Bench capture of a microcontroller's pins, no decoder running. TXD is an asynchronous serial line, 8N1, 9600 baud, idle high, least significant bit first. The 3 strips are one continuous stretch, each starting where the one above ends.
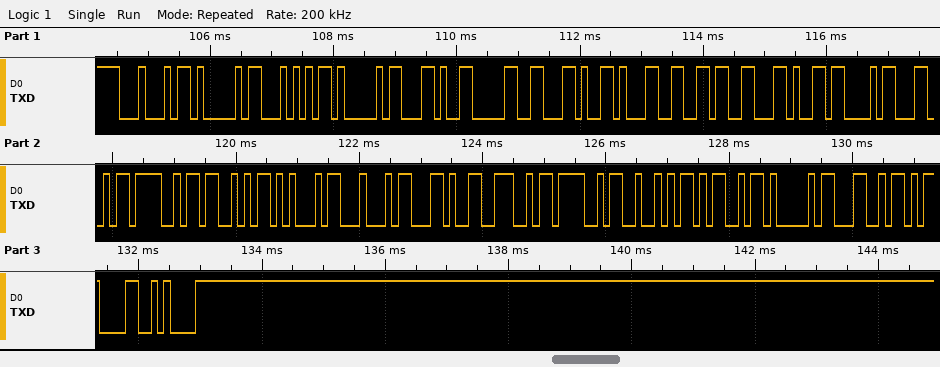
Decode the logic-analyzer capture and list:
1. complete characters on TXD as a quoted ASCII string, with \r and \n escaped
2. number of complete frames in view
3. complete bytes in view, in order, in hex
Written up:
"DATA,0,16,CLOSED,NORMAL\r\n"
25
44 41 54 41 2C 30 2C 31 36 2C 43 4C 4F 53 45 44 2C 4E 4F 52 4D 41 4C 0D 0A
